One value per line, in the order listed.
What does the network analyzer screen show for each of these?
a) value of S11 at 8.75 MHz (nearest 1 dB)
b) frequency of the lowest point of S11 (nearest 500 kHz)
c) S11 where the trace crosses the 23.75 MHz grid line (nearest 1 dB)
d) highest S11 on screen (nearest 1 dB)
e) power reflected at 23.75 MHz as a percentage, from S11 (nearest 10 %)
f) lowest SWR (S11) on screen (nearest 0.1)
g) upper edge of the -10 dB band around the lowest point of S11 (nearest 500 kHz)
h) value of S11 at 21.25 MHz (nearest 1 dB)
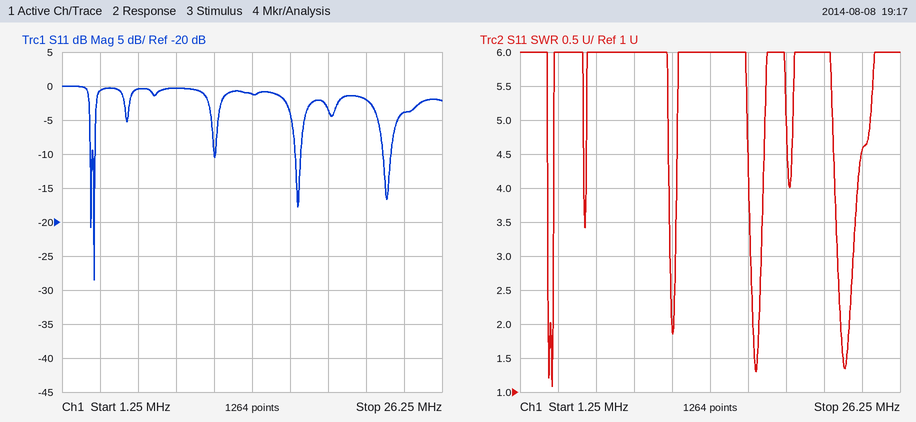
0 dB
3.5 MHz
-4 dB
0 dB
40 %
1.1
3.5 MHz
-2 dB
